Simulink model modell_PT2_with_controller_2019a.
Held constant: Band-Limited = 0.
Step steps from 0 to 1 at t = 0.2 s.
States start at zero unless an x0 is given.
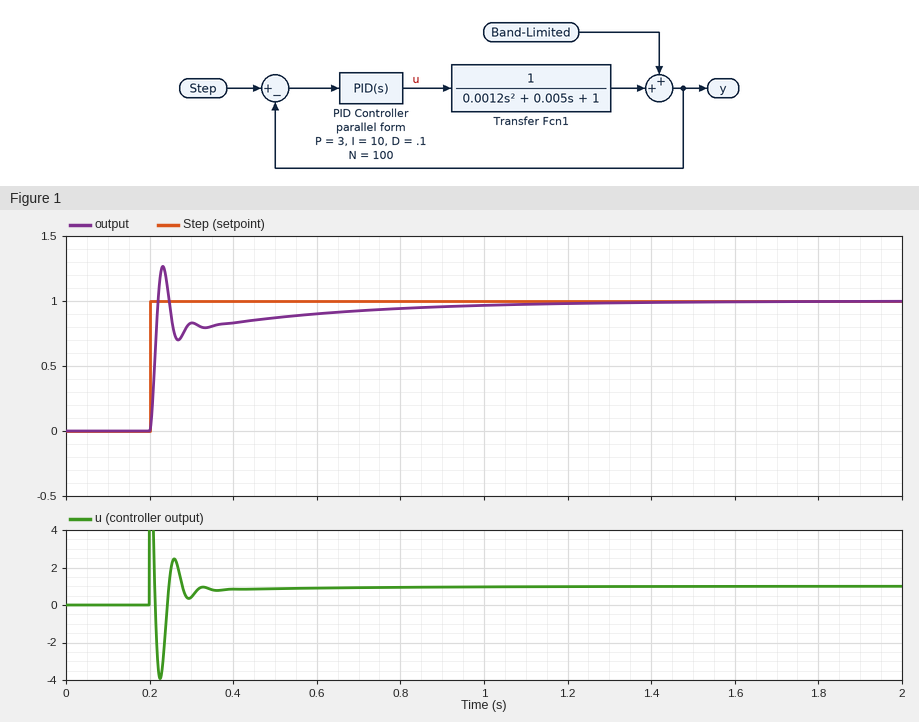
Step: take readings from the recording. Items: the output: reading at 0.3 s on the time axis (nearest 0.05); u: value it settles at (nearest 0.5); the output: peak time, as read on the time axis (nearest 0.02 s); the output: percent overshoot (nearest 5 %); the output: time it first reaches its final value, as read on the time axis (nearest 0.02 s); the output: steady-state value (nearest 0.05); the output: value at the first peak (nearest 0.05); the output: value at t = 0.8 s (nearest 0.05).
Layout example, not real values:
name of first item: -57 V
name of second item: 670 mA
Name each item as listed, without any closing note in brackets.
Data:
the output: reading at 0.3 s on the time axis: 0.85
u: value it settles at: 1.0
the output: peak time, as read on the time axis: 0.24 s
the output: percent overshoot: 25 %
the output: time it first reaches its final value, as read on the time axis: 0.22 s
the output: steady-state value: 1.00
the output: value at the first peak: 1.25
the output: value at t = 0.8 s: 0.95
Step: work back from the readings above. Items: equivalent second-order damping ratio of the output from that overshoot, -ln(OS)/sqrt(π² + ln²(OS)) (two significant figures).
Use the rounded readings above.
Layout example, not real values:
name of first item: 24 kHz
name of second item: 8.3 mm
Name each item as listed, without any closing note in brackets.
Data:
equivalent second-order damping ratio of the output from that overshoot, -ln(OS)/sqrt(π² + ln²(OS)): 0.40
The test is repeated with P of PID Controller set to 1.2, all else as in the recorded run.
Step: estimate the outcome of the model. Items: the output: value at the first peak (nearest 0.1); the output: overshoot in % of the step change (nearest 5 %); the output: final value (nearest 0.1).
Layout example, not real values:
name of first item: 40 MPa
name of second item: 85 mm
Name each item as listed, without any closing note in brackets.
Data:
the output: value at the first peak: 1.1
the output: overshoot in % of the step change: 10 %
the output: final value: 1.0
